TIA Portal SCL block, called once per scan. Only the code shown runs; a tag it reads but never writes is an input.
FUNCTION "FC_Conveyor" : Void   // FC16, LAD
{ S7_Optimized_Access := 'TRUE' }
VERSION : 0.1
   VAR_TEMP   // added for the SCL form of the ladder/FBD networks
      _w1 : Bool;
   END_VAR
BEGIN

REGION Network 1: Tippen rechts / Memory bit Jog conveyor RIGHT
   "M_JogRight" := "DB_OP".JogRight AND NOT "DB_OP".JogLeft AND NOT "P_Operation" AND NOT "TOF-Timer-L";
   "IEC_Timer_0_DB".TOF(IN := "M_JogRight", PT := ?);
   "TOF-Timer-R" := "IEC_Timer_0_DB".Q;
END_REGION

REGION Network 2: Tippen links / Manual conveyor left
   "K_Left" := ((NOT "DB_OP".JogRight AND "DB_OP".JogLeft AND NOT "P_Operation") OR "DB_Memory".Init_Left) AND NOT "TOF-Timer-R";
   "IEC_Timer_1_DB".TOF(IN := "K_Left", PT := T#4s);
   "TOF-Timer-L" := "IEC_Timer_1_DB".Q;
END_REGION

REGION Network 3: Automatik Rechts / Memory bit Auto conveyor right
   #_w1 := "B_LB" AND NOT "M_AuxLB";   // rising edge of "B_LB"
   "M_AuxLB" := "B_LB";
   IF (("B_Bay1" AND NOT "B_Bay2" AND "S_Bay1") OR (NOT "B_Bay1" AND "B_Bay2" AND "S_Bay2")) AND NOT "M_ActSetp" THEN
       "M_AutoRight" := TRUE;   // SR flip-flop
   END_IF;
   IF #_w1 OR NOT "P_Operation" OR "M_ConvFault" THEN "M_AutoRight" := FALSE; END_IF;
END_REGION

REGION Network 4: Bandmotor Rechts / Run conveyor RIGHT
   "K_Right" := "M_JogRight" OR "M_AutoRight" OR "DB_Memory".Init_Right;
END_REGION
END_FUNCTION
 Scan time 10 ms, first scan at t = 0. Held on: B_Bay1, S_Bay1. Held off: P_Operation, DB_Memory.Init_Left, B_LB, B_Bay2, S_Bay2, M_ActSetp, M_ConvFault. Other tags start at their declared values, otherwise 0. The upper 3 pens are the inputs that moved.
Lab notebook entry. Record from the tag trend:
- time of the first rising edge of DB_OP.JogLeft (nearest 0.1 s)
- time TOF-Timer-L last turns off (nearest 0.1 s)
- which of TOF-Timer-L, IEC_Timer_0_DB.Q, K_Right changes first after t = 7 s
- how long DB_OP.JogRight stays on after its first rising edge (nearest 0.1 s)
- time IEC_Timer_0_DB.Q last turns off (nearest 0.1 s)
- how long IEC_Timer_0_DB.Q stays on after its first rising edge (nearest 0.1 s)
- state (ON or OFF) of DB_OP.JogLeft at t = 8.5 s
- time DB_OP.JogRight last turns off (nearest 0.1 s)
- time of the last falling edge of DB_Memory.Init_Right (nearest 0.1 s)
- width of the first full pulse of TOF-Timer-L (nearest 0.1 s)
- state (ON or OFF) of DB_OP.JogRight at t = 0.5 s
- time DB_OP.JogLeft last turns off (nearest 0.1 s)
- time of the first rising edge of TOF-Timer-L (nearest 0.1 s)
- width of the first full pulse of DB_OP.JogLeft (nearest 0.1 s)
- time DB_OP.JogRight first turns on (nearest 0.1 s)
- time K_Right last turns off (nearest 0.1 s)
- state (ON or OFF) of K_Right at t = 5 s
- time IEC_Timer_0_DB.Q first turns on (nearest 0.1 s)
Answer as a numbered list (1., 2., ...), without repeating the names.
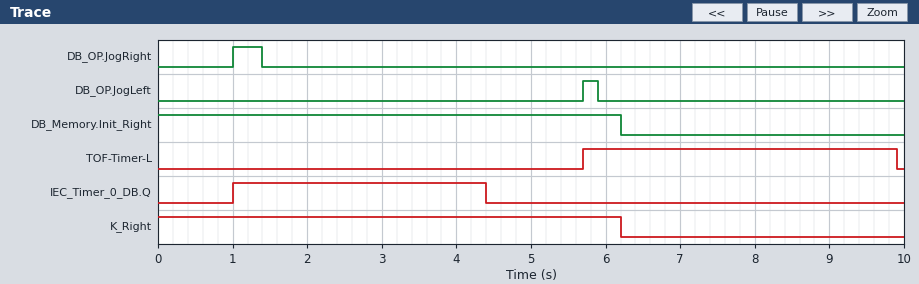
1. 5.7 s
2. 9.9 s
3. TOF-Timer-L
4. 0.4 s
5. 4.4 s
6. 3.4 s
7. OFF
8. 1.4 s
9. 6.2 s
10. 4.2 s
11. OFF
12. 5.9 s
13. 5.7 s
14. 0.2 s
15. 1.0 s
16. 6.2 s
17. ON
18. 1.0 s
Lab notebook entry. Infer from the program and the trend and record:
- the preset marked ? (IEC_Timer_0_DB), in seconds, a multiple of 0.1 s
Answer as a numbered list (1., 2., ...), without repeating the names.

1. 3.0 s
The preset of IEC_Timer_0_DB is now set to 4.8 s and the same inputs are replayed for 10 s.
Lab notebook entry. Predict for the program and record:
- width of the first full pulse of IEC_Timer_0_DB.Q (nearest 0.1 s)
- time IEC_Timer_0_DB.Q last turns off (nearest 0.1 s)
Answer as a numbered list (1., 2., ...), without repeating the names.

1. 5.2 s
2. 6.2 s
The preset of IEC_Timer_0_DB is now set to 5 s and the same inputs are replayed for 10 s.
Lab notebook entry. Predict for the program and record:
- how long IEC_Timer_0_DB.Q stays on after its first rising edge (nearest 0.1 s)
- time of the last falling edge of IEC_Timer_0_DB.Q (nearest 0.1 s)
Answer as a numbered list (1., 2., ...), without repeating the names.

1. 5.4 s
2. 6.4 s
